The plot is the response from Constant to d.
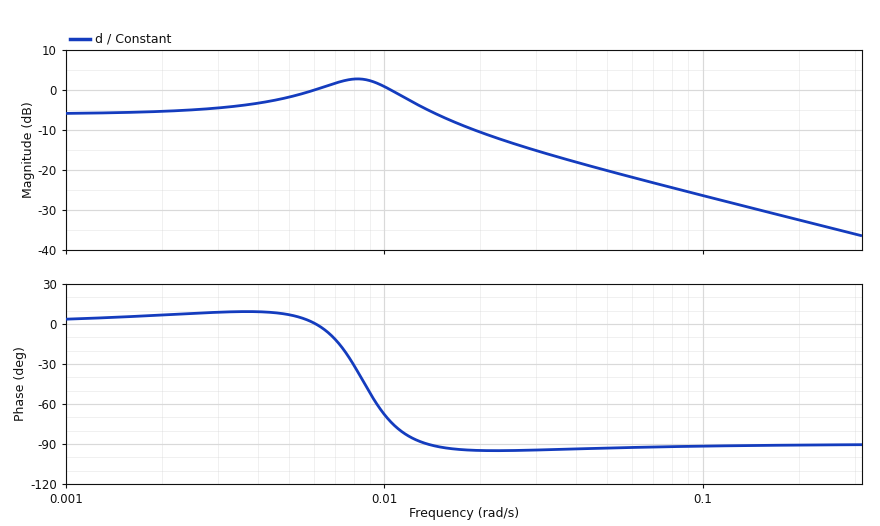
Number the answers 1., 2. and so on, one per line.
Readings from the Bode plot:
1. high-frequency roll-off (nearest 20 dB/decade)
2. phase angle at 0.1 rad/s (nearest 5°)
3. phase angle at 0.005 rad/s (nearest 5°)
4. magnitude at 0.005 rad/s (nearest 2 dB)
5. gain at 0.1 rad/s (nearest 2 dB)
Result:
1. -20 dB/decade
2. -90°
3. 5°
4. -2 dB
5. -26 dB
